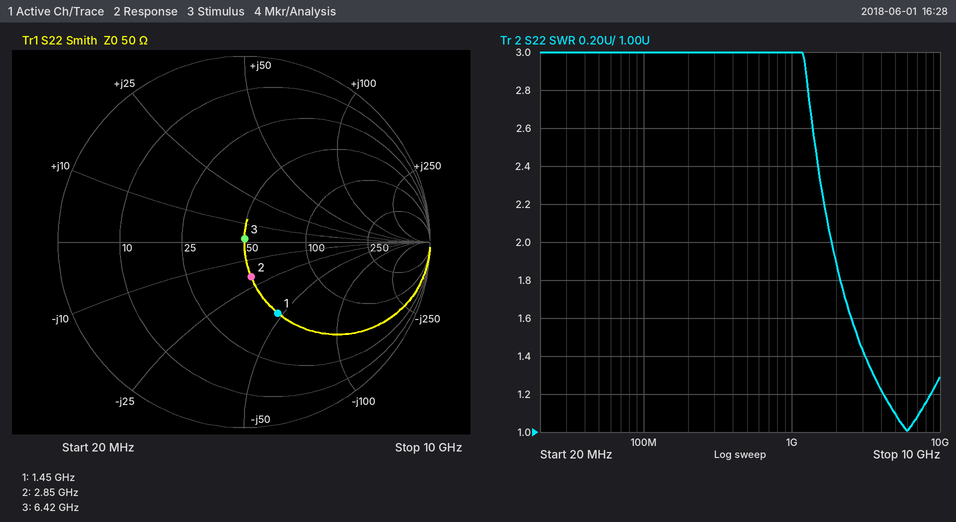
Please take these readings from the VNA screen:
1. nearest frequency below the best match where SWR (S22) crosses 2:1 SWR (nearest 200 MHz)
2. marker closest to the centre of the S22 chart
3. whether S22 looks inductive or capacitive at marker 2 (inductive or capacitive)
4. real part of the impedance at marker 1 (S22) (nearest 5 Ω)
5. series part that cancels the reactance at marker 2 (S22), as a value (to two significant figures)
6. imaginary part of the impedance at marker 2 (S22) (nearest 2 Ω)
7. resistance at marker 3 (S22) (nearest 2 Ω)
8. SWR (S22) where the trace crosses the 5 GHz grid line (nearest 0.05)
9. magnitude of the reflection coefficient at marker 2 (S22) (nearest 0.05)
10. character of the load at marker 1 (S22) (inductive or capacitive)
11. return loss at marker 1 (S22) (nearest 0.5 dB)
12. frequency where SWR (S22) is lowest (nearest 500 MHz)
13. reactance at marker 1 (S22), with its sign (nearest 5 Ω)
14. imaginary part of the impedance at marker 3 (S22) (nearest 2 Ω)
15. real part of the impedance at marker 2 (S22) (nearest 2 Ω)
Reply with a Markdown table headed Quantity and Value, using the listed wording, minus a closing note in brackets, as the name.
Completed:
| Quantity | Value |
|---|---|
| nearest frequency below the best match where SWR (S22) crosses 2:1 SWR | 1.8 GHz |
| marker closest to the centre of the S22 chart | marker 3 |
| whether S22 looks inductive or capacitive at marker 2 | capacitive |
| real part of the impedance at marker 1 (S22) | 50 Ω |
| series part that cancels the reactance at marker 2 (S22), as a value | 1.1 nH |
| imaginary part of the impedance at marker 2 (S22) | -20 Ω |
| resistance at marker 3 (S22) | 50 Ω |
| SWR (S22) where the trace crosses the 5 GHz grid line | 1.10 |
| magnitude of the reflection coefficient at marker 2 (S22) | 0.20 |
| character of the load at marker 1 (S22) | capacitive |
| return loss at marker 1 (S22) | 7.5 dB |
| frequency where SWR (S22) is lowest | 6.0 GHz |
| reactance at marker 1 (S22), with its sign | -45 Ω |
| imaginary part of the impedance at marker 3 (S22) | +2 Ω |
| real part of the impedance at marker 2 (S22) | 50 Ω |
